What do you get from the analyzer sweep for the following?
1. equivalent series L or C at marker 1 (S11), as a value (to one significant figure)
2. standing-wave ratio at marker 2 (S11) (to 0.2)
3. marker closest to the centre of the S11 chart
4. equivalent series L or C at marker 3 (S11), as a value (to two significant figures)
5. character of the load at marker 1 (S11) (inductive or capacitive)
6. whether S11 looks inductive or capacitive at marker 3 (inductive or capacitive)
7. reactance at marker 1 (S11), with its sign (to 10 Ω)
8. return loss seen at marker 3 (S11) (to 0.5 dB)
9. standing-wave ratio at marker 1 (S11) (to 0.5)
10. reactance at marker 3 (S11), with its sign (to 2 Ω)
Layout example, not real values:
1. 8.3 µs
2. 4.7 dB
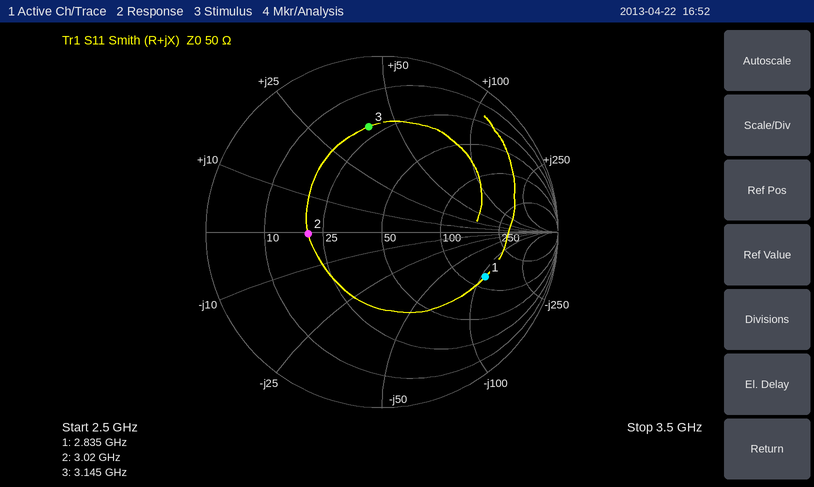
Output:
1. 500 fF
2. 2.4
3. marker 2
4. 2.0 nH
5. capacitive
6. inductive
7. -110 Ω
8. 4.5 dB
9. 4.5
10. +40 Ω
